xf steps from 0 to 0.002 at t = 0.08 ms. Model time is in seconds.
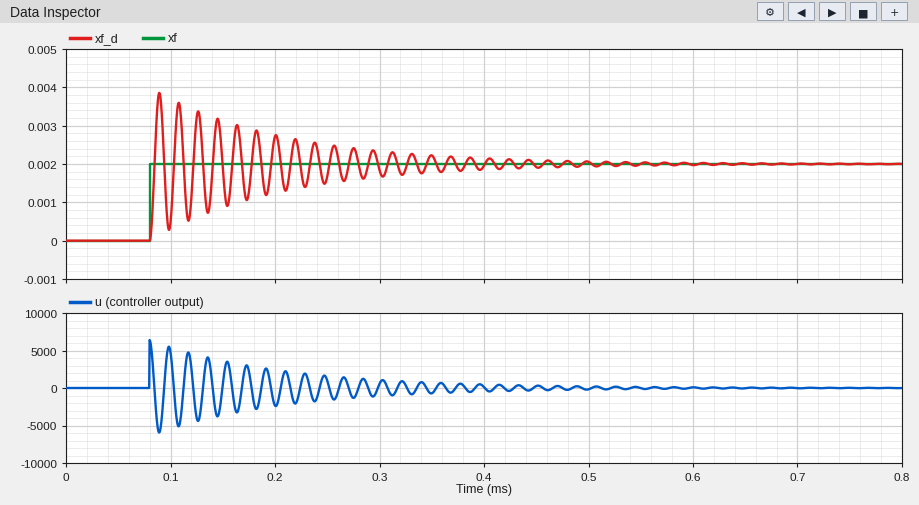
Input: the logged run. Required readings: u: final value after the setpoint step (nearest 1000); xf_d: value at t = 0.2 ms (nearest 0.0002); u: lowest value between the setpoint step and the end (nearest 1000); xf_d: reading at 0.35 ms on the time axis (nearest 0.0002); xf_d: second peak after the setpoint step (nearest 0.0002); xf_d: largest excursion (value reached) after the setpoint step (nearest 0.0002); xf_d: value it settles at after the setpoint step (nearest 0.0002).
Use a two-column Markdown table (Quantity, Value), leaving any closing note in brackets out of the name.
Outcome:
| Quantity | Value |
|---|---|
| u: final value after the setpoint step | 0 |
| xf_d: value at t = 0.2 ms | 0.0028 |
| u: lowest value between the setpoint step and the end | -6000 |
| xf_d: reading at 0.35 ms on the time axis | 0.0022 |
| xf_d: second peak after the setpoint step | 0.0036 |
| xf_d: largest excursion (value reached) after the setpoint step | 0.0038 |
| xf_d: value it settles at after the setpoint step | 0.0020 |
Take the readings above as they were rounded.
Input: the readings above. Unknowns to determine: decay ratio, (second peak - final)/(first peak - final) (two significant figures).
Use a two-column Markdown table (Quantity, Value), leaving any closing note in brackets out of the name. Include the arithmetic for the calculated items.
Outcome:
| Quantity | Value |
|---|---|
| decay ratio, (second peak - final)/(first peak - final) | (0.0036 - 0.002) / (0.0038 - 0.002) = 0.89 |
